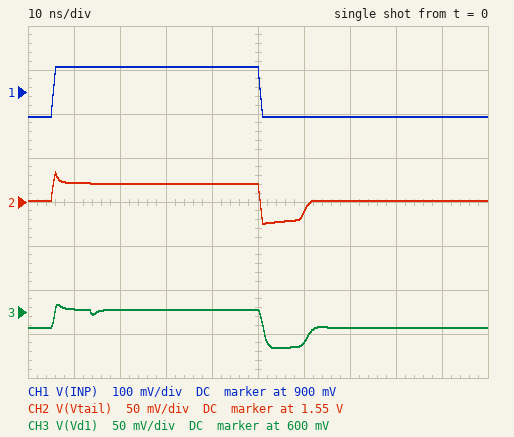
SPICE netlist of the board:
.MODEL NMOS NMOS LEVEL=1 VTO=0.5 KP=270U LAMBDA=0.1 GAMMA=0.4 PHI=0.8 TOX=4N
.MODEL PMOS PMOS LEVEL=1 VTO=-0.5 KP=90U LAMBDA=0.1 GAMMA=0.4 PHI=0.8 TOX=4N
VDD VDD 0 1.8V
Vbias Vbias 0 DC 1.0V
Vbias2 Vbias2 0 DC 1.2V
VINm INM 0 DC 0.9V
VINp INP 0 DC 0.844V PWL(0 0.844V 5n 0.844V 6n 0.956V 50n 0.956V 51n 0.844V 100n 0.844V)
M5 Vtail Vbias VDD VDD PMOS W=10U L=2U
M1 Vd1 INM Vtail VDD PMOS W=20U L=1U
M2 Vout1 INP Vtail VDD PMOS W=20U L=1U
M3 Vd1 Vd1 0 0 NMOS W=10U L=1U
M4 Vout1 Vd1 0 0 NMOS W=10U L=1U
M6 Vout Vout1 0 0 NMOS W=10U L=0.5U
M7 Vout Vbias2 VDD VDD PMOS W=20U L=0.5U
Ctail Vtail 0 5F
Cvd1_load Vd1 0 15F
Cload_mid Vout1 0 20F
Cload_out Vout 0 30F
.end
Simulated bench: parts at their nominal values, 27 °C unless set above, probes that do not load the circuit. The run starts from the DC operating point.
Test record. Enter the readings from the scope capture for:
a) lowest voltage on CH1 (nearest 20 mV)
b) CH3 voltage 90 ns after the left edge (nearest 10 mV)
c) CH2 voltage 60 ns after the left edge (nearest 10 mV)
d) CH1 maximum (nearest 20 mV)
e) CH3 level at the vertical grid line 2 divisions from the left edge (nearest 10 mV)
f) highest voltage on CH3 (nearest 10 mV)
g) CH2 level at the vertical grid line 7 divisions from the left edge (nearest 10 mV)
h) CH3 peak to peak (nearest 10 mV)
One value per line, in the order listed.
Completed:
840 mV
580 mV
1.54 V
960 mV
600 mV
610 mV
1.55 V
50 mV
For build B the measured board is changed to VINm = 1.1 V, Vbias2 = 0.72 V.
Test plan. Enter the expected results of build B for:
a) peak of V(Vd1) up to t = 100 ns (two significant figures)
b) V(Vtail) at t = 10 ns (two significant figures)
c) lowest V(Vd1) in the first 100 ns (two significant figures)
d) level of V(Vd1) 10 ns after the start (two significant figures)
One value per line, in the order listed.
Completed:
580 mV
1.7 V
540 mV
560 mV
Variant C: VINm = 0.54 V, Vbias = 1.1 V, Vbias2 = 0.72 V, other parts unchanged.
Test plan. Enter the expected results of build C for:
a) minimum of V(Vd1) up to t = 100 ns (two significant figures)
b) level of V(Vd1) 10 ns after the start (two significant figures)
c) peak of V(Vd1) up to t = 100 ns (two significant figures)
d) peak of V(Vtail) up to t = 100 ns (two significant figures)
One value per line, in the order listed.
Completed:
570 mV
580 mV
590 mV
1.3 V
